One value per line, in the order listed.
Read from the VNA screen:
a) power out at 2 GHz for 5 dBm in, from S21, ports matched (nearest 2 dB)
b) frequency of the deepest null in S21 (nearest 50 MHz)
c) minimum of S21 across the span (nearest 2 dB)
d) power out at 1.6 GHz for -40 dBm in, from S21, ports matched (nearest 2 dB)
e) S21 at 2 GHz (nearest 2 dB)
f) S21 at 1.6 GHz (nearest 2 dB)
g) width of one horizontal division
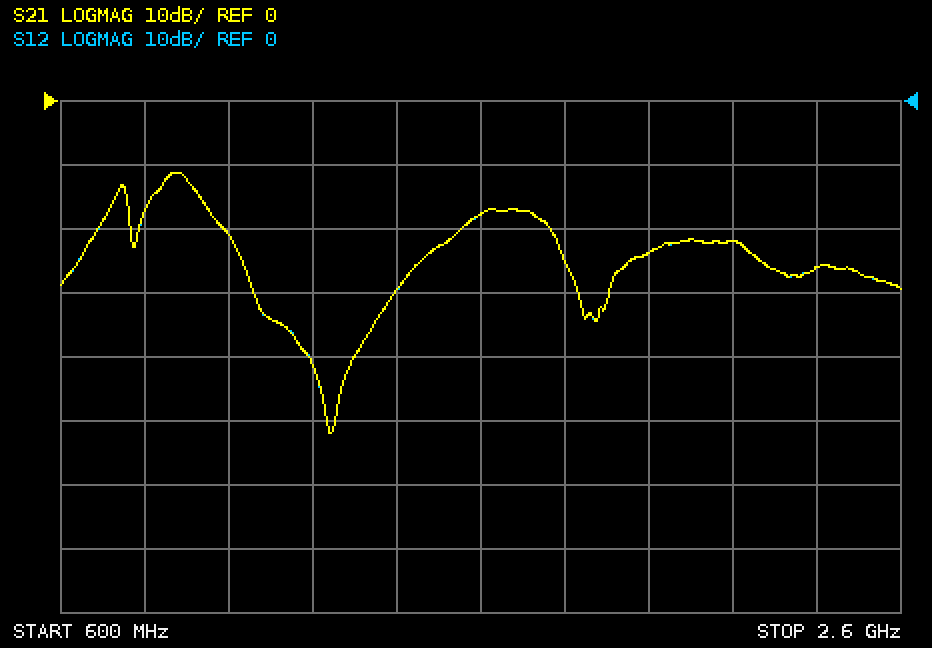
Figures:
-18 dBm
1.25 GHz
-52 dB
-58 dBm
-24 dB
-18 dB
200 MHz
